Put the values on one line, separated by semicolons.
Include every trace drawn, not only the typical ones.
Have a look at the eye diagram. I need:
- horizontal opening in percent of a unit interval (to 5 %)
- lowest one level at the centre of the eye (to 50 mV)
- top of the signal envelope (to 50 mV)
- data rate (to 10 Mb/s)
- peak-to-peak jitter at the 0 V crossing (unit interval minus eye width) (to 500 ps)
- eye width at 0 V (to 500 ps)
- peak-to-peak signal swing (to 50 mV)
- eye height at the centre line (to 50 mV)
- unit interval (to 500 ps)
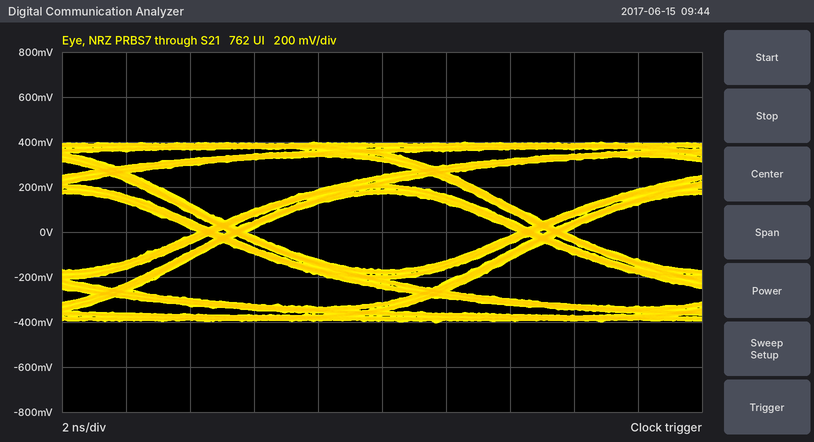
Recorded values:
85 %; 150 mV; 400 mV; 100 Mb/s; 1.5 ns; 8.5 ns; 800 mV; 350 mV; 10.0 ns
